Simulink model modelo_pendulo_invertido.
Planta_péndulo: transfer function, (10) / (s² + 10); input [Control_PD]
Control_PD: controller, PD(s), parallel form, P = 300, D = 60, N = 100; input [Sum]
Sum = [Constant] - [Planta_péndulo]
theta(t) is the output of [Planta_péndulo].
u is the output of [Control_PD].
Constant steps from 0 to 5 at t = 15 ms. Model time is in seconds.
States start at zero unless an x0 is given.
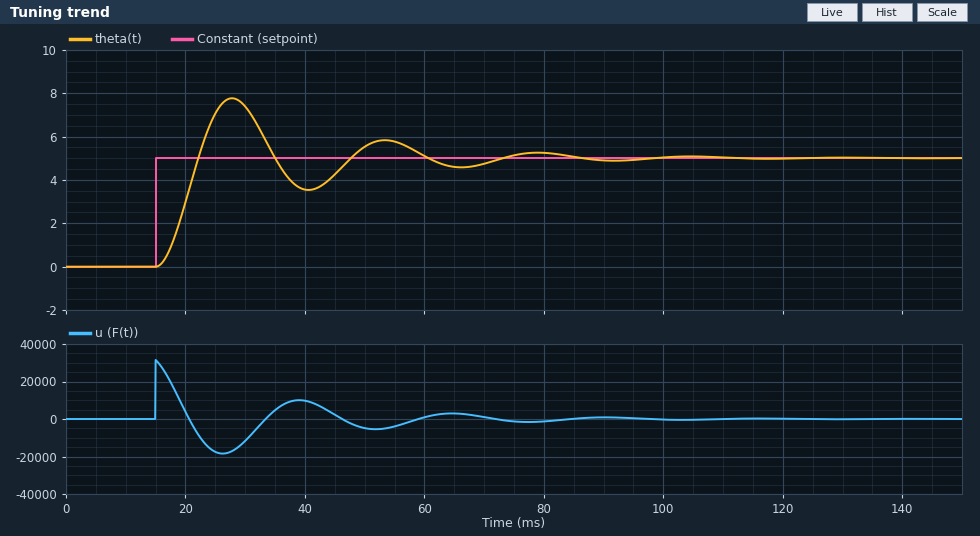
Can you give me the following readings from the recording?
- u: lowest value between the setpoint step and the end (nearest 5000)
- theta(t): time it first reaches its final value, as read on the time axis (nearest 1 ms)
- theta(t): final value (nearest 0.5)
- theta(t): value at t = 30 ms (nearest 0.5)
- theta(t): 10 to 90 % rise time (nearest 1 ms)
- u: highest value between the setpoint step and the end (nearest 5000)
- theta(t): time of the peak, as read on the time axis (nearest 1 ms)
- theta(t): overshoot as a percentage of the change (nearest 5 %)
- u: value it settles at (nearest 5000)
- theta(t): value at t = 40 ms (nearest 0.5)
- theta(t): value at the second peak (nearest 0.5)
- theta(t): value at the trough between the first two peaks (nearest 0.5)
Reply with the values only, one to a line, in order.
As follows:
-20000
22 ms
5.0
7.5
5 ms
30000
28 ms
55 %
0
3.5
6.0
3.5
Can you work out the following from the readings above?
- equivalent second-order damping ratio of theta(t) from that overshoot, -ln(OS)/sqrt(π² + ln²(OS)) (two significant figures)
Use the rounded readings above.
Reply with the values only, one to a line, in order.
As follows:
0.19
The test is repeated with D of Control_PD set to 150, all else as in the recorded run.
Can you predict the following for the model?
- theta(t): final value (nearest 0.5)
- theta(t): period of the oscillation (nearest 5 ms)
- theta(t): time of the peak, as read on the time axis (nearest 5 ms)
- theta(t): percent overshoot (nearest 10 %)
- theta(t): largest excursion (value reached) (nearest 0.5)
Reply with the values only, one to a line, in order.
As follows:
5.0
15 ms
25 ms
70 %
8.5
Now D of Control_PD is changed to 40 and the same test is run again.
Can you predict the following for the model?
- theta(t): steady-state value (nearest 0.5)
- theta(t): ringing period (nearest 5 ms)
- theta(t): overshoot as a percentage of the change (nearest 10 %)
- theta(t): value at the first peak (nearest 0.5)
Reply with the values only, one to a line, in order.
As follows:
5.0
30 ms
50 %
7.5
